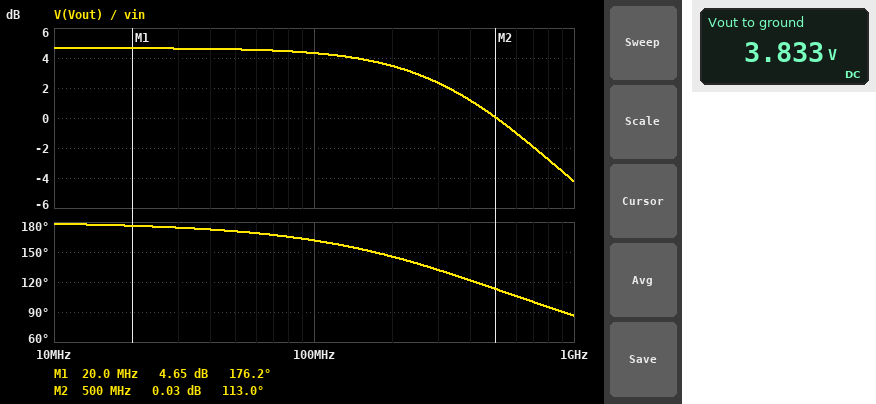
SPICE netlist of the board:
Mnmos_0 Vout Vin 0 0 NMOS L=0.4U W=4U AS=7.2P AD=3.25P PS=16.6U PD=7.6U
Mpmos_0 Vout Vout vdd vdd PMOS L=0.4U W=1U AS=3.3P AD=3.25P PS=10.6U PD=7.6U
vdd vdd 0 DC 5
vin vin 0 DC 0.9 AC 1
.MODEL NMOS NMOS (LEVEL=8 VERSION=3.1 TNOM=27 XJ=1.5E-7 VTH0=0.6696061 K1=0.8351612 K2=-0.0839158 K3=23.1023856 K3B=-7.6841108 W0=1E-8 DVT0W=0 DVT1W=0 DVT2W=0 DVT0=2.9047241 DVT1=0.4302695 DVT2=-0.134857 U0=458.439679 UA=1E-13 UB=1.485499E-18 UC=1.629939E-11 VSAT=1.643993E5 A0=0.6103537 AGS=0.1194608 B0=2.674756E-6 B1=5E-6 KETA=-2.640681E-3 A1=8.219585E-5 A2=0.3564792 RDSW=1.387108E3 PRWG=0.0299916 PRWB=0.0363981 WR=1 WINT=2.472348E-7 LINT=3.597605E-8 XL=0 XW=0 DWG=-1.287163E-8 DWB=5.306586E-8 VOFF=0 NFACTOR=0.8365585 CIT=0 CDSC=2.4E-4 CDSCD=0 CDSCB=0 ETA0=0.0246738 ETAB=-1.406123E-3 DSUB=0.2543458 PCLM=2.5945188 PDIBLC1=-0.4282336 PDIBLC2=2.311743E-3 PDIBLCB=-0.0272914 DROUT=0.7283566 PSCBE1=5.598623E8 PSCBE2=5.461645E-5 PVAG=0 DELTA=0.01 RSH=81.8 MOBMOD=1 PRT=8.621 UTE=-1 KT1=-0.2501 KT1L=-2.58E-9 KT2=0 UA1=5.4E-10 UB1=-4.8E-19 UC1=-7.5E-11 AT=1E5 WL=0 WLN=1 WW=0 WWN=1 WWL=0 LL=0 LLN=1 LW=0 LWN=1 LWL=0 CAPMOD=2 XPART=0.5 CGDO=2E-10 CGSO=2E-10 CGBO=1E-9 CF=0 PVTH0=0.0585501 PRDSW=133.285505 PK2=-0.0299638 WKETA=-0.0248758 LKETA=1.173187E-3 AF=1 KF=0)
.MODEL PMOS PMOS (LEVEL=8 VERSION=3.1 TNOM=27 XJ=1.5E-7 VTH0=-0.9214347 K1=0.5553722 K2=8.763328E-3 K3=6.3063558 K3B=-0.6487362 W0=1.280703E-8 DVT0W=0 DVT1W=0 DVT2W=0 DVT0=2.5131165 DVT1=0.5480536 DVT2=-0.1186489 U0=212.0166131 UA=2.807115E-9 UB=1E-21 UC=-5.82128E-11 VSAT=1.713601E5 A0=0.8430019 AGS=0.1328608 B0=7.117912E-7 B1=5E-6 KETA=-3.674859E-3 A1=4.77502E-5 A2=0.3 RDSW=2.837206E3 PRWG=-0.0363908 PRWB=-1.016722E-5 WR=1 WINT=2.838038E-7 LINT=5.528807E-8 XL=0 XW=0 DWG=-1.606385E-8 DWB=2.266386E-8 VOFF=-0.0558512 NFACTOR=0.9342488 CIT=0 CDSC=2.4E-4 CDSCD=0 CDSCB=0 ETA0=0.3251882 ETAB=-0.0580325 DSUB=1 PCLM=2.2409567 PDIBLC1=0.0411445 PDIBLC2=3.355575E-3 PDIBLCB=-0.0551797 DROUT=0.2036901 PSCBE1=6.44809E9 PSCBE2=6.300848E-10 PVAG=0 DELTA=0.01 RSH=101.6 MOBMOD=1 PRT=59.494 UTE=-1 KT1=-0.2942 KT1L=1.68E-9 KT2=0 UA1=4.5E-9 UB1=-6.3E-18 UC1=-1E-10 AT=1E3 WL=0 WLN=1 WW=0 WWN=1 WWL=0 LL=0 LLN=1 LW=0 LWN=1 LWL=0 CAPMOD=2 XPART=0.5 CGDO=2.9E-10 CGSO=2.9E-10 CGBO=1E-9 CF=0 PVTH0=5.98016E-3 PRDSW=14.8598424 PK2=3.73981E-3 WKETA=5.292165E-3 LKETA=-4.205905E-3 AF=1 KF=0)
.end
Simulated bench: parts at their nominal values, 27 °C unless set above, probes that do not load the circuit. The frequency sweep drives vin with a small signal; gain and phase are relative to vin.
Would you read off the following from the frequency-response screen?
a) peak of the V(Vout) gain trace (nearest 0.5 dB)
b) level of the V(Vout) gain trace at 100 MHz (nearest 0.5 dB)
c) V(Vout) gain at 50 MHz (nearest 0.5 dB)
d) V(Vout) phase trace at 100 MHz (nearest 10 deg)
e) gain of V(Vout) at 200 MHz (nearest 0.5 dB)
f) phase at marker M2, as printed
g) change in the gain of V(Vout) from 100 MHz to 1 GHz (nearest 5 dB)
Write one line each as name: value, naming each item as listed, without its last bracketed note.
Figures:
peak of the V(Vout) gain trace: 4.5 dB
level of the V(Vout) gain trace at 100 MHz: 4.5 dB
V(Vout) gain at 50 MHz: 4.5 dB
V(Vout) phase trace at 100 MHz: 160 deg
gain of V(Vout) at 200 MHz: 3.5 dB
phase at marker M2, as printed: 113.0 deg
change in the gain of V(Vout) from 100 MHz to 1 GHz: -10 dB
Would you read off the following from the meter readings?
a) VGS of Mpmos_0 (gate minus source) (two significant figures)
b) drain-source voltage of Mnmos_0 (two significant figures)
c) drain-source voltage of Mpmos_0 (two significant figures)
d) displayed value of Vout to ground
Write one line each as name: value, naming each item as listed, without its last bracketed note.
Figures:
VGS of Mpmos_0 (gate minus source): -1.2 V
drain-source voltage of Mnmos_0: 3.8 V
drain-source voltage of Mpmos_0: -1.2 V
displayed value of Vout to ground: 3.833 V
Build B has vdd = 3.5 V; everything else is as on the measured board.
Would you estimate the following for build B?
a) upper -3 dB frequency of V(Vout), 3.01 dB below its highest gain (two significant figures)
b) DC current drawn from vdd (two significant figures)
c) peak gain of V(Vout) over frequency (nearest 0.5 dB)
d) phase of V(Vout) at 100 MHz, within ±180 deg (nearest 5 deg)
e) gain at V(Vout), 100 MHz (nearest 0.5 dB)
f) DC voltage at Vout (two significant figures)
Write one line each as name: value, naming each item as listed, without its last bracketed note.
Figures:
upper -3 dB frequency of V(Vout), 3.01 dB below its highest gain: 110 MHz
DC current drawn from vdd: 240 nA
peak gain of V(Vout) over frequency: 1.5 dB
phase of V(Vout) at 100 MHz, within ±180 deg: 125 deg
gain at V(Vout), 100 MHz: -1.0 dB
DC voltage at Vout: 2.4 V
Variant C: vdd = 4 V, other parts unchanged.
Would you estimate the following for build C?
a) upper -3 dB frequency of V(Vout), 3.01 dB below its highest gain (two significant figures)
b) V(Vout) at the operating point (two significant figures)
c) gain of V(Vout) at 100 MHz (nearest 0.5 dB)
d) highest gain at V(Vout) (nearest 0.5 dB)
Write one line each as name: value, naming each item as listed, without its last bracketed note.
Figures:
upper -3 dB frequency of V(Vout), 3.01 dB below its highest gain: 150 MHz
V(Vout) at the operating point: 2.9 V
gain of V(Vout) at 100 MHz: 0.5 dB
highest gain at V(Vout): 2.0 dB
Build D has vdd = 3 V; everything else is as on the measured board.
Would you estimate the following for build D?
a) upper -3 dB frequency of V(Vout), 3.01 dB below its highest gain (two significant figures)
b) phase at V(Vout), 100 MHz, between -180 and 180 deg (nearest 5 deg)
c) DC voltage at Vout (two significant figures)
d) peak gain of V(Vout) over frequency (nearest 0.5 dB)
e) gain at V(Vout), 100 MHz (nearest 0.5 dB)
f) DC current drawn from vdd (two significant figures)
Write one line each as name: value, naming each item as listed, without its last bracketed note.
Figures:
upper -3 dB frequency of V(Vout), 3.01 dB below its highest gain: 95 MHz
phase at V(Vout), 100 MHz, between -180 and 180 deg: 120 deg
DC voltage at Vout: 1.9 V
peak gain of V(Vout) over frequency: 1.5 dB
gain at V(Vout), 100 MHz: -1.5 dB
DC current drawn from vdd: 210 nA
